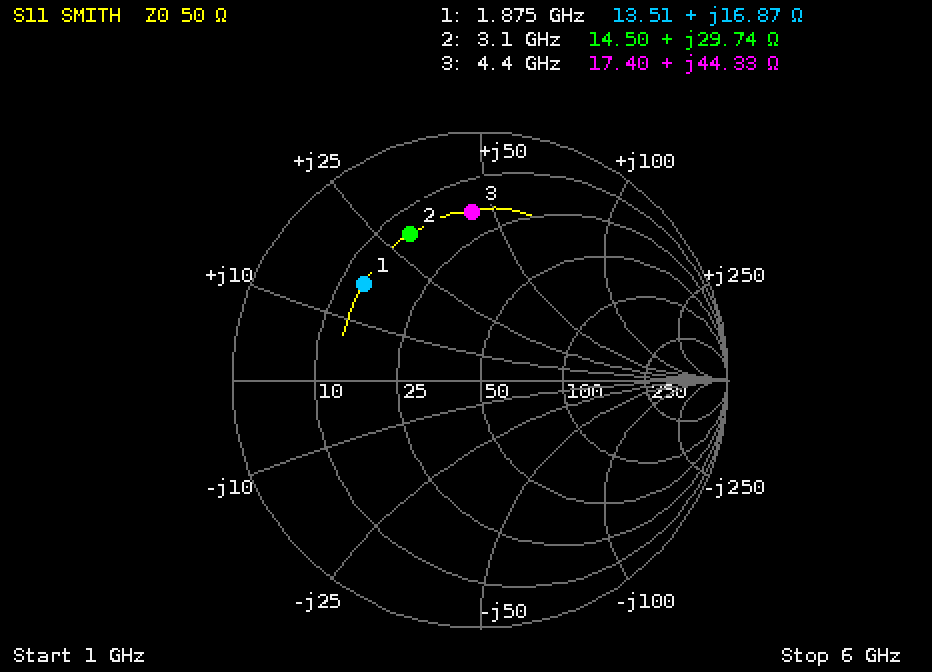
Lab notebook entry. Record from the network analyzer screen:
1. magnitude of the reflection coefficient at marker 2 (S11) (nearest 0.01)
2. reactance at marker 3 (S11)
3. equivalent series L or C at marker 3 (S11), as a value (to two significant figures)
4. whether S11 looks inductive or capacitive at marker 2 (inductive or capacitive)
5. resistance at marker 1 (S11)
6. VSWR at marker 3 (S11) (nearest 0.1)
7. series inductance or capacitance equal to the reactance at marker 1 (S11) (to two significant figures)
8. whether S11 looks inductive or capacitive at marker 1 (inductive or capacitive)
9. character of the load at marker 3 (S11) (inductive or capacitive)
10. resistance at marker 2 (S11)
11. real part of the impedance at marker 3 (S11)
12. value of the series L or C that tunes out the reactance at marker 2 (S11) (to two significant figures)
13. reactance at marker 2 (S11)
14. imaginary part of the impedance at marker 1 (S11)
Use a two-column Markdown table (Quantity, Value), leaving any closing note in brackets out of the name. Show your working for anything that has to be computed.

| Quantity | Value |
|---|---|
| magnitude of the reflection coefficient at marker 2 (S11) | 0.65 |
| reactance at marker 3 | +44.33 Ω |
| equivalent series L or C at marker 3 (S11), as a value | L = 44.33 Ω/(2π × 4.4 GHz) ≈ 1.6 nH |
| whether S11 looks inductive or capacitive at marker 2 | inductive |
| resistance at marker 1 | 13.51 Ω |
| VSWR at marker 3 (S11) | 5.3 |
| series inductance or capacitance equal to the reactance at marker 1 (S11) | L = 16.87 Ω/(2π × 1.875 GHz) ≈ 1.4 nH |
| whether S11 looks inductive or capacitive at marker 1 | inductive |
| character of the load at marker 3 (S11) | inductive |
| resistance at marker 2 | 14.50 Ω |
| real part of the impedance at marker 3 | 17.40 Ω |
| value of the series L or C that tunes out the reactance at marker 2 (S11) | C = 1/(2π × 3.1 GHz × 29.74 Ω) ≈ 1.7 pF |
| reactance at marker 2 | +29.74 Ω |
| imaginary part of the impedance at marker 1 | +16.87 Ω |
